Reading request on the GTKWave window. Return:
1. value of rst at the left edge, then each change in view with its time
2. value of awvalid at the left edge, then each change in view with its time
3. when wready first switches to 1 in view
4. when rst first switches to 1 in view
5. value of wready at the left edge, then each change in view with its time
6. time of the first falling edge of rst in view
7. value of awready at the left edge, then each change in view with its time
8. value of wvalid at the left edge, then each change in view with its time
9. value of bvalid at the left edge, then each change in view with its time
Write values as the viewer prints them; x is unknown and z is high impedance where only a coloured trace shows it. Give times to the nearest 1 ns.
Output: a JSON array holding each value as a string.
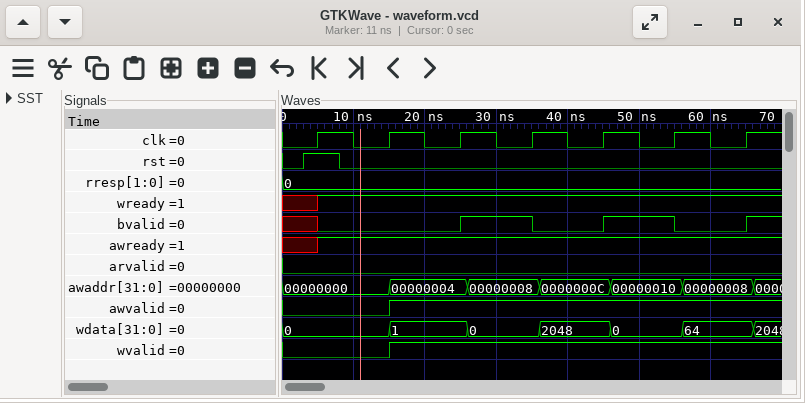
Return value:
["0, 1 at 3 ns, 0 at 8 ns", "0, 1 at 15 ns", "5 ns", "3 ns", "x, 1 at 5 ns", "8 ns", "x, 1 at 5 ns", "0, 1 at 15 ns", "x, 0 at 5 ns, 1 at 25 ns, 0 at 35 ns, 1 at 45 ns, 0 at 55 ns, 1 at 65 ns"]
